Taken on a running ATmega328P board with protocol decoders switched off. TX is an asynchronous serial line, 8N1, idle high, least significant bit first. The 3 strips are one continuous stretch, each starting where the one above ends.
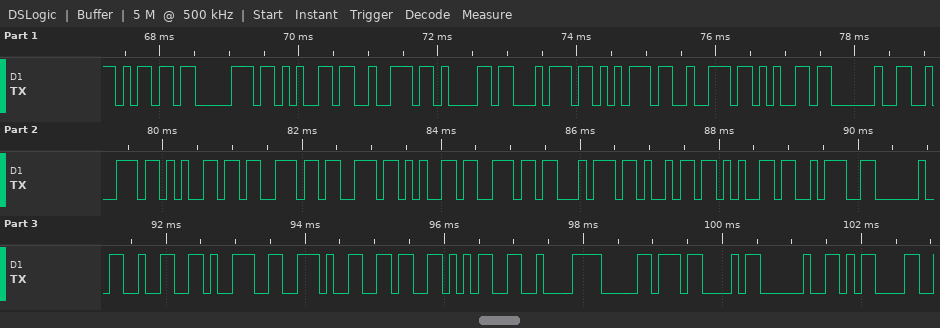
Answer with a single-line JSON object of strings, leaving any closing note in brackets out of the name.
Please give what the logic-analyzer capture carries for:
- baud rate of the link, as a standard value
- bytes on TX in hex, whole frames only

{"baud rate of the link, as a standard value": "9600 baud", "bytes on TX in hex, whole frames only": "0x6D 0x70 0x65 0x72 0x61 0x74 0x75 0x72 0x65 0x20 0x72 0x65 0x73 0x73 0x65 0x6E 0x74 0x69 0x65 0x3A 0x20 0x32 0x39 0x2E 0x36 0x35 0xC2 0xB0 0x43 0x20 0x0D"}
